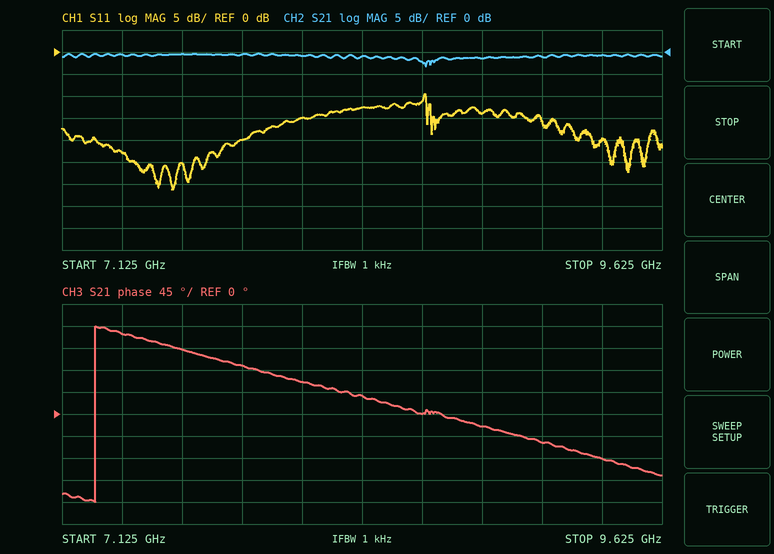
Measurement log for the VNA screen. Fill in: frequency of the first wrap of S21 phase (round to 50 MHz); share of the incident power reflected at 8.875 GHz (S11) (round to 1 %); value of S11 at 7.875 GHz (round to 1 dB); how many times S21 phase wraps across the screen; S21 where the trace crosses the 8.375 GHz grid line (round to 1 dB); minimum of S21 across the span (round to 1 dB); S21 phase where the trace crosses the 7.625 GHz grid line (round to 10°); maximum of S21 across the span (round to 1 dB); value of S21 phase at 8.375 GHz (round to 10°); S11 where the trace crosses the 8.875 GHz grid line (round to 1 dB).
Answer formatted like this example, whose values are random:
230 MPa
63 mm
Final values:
7.25 GHz
4 %
-20 dB
1
-1 dB
-3 dB
130°
0 dB
40°
-14 dB
